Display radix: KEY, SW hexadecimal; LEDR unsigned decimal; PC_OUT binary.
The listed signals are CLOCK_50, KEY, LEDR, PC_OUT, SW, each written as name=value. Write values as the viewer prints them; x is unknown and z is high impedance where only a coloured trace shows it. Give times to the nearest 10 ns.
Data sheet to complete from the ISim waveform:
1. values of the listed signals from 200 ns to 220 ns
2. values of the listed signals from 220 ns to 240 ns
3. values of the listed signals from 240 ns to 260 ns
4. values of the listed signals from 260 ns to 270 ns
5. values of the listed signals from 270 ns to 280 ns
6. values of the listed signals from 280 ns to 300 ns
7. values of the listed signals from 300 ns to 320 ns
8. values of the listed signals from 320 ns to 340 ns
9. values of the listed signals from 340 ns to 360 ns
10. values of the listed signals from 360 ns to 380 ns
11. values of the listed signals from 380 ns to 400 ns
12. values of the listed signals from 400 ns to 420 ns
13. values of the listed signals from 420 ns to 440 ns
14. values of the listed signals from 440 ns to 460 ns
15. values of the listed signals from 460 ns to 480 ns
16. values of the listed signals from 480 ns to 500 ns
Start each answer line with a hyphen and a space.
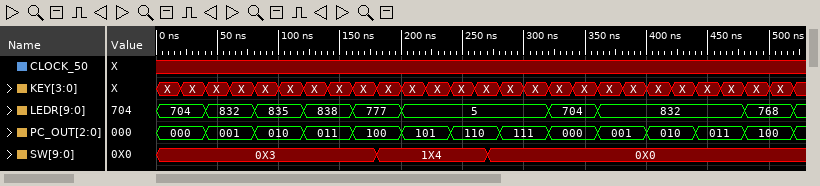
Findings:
- CLOCK_50=x, KEY=X, LEDR=5, PC_OUT=101, SW=1X4
- CLOCK_50=x, KEY=X, LEDR=5, PC_OUT=101, SW=1X4
- CLOCK_50=x, KEY=X, LEDR=5, PC_OUT=110, SW=1X4
- CLOCK_50=x, KEY=X, LEDR=5, PC_OUT=110, SW=1X4
- CLOCK_50=x, KEY=X, LEDR=5, PC_OUT=110, SW=0X0
- CLOCK_50=x, KEY=X, LEDR=5, PC_OUT=111, SW=0X0
- CLOCK_50=x, KEY=X, LEDR=5, PC_OUT=111, SW=0X0
- CLOCK_50=x, KEY=X, LEDR=704, PC_OUT=000, SW=0X0
- CLOCK_50=x, KEY=X, LEDR=704, PC_OUT=000, SW=0X0
- CLOCK_50=x, KEY=X, LEDR=832, PC_OUT=001, SW=0X0
- CLOCK_50=x, KEY=X, LEDR=832, PC_OUT=001, SW=0X0
- CLOCK_50=x, KEY=X, LEDR=832, PC_OUT=010, SW=0X0
- CLOCK_50=x, KEY=X, LEDR=832, PC_OUT=010, SW=0X0
- CLOCK_50=x, KEY=X, LEDR=832, PC_OUT=011, SW=0X0
- CLOCK_50=x, KEY=X, LEDR=832, PC_OUT=011, SW=0X0
- CLOCK_50=x, KEY=X, LEDR=768, PC_OUT=100, SW=0X0
